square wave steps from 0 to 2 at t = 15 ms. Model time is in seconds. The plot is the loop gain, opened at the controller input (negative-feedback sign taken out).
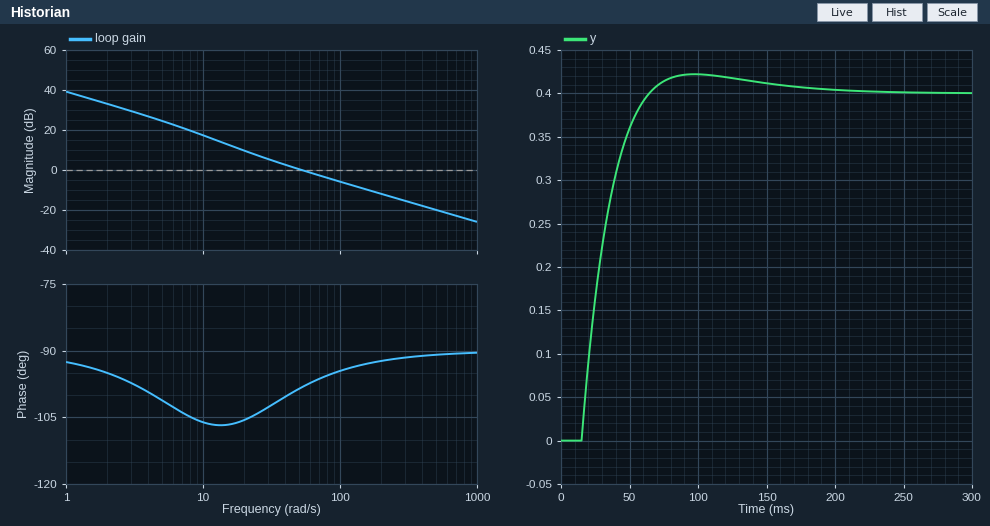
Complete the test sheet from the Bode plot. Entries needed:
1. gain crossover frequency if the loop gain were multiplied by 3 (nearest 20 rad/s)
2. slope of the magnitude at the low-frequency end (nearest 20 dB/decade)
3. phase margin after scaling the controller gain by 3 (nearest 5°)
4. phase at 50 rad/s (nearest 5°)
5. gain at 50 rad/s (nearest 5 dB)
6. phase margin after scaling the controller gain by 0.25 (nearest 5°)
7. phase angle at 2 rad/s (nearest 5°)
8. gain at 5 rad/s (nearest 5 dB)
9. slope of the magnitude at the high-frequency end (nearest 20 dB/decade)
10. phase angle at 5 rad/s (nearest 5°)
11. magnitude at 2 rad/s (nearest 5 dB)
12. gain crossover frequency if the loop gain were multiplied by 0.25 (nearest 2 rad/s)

160 rad/s
-20 dB/decade
85°
-100°
0 dB
75°
-95°
25 dB
-20 dB/decade
-100°
35 dB
16 rad/s
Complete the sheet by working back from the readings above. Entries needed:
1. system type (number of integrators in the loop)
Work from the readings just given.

1
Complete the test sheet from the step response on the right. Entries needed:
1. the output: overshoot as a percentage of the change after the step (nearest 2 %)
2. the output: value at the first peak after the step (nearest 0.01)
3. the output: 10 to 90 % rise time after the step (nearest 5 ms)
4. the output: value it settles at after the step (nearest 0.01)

6 %
0.42
35 ms
0.40
